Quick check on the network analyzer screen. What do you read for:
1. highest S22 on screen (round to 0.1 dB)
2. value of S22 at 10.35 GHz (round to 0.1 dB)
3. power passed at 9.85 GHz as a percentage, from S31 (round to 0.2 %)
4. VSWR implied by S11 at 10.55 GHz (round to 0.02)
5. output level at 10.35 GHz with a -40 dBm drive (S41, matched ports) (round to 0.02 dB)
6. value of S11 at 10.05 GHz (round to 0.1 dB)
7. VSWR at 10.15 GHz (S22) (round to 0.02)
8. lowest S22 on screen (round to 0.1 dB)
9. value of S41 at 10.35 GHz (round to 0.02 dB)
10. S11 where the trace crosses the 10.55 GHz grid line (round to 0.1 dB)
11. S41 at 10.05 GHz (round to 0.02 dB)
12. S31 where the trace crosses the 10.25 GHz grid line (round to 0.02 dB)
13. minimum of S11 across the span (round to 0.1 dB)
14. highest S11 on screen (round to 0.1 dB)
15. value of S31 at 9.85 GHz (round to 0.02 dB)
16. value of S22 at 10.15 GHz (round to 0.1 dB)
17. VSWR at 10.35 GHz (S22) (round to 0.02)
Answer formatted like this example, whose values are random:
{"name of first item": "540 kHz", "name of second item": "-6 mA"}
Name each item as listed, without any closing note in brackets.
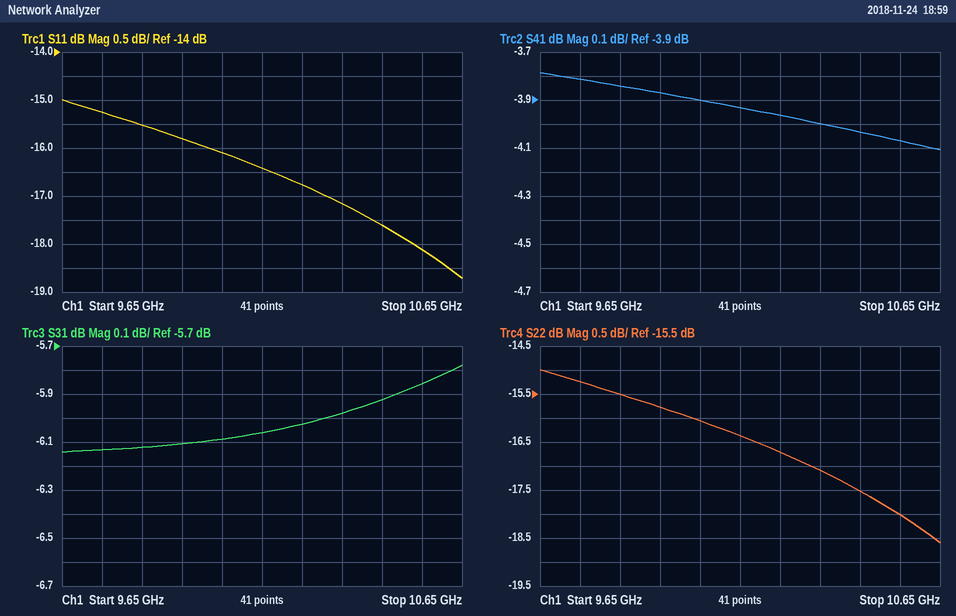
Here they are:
{"highest S22 on screen": "-15.0 dB", "value of S22 at 10.35 GHz": "-17.1 dB", "power passed at 9.85 GHz as a percentage, from S31": "24.4 %", "VSWR implied by S11 at 10.55 GHz": "1.28", "output level at 10.35 GHz with a -40 dBm drive (S41, matched ports)": "-44.00 dBm", "value of S11 at 10.05 GHz": "-16.1 dB", "VSWR at 10.15 GHz (S22)": "1.36", "lowest S22 on screen": "-18.6 dB", "value of S41 at 10.35 GHz": "-4.00 dB", "S11 where the trace crosses the 10.55 GHz grid line": "-18.1 dB", "S41 at 10.05 GHz": "-3.90 dB", "S31 where the trace crosses the 10.25 GHz grid line": "-6.02 dB", "minimum of S11 across the span": "-18.7 dB", "highest S11 on screen": "-15.0 dB", "value of S31 at 9.85 GHz": "-6.12 dB", "value of S22 at 10.15 GHz": "-16.4 dB", "VSWR at 10.35 GHz (S22)": "1.32"}
